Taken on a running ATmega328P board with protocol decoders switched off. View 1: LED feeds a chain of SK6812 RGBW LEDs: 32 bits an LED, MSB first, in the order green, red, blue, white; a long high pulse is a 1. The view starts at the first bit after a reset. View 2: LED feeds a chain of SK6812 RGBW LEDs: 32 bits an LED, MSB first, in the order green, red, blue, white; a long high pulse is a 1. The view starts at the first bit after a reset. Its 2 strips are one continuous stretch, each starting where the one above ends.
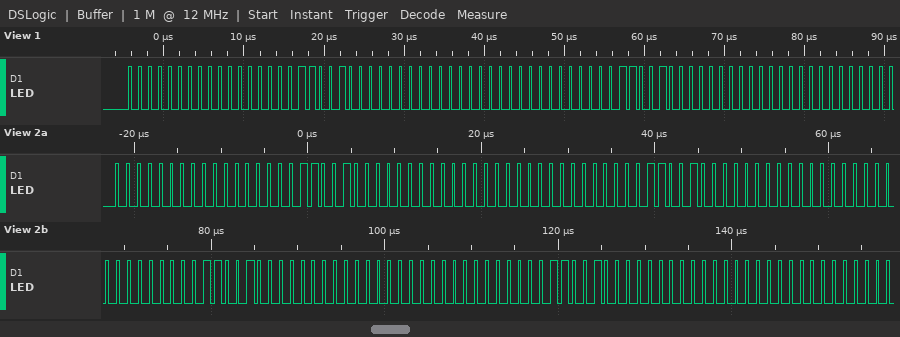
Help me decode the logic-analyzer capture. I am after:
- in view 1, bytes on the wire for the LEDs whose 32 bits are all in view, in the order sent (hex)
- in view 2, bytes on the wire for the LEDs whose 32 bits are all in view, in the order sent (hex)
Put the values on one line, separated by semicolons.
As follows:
00 00 64 00 00 00 64 00; 00 00 64 00 00 00 64 00 00 00 64 00 00 00 64 00
